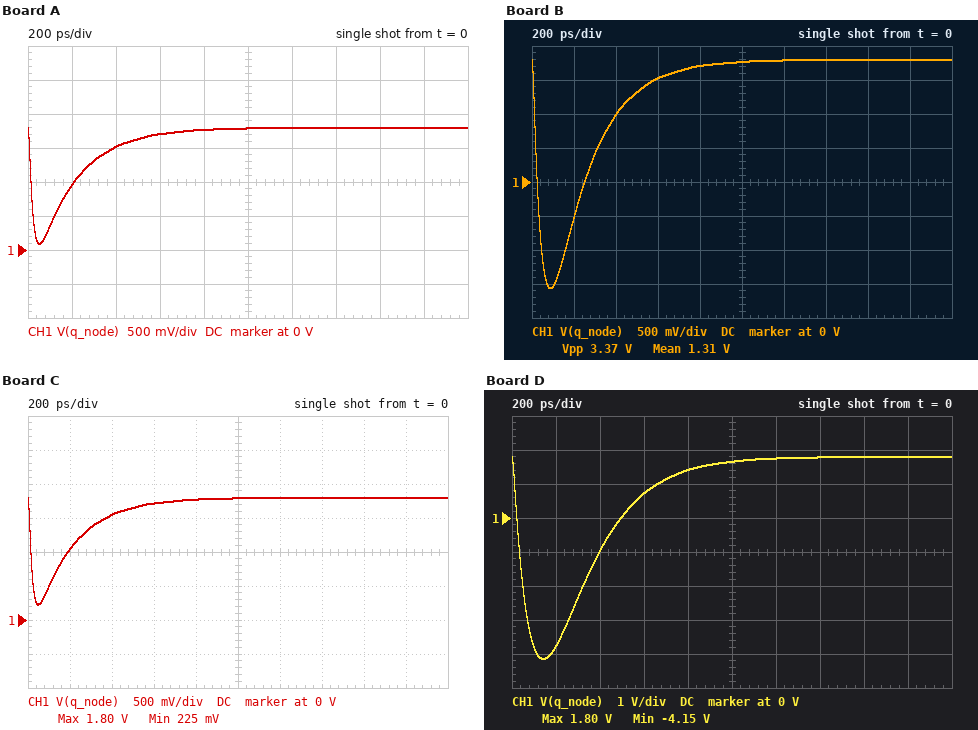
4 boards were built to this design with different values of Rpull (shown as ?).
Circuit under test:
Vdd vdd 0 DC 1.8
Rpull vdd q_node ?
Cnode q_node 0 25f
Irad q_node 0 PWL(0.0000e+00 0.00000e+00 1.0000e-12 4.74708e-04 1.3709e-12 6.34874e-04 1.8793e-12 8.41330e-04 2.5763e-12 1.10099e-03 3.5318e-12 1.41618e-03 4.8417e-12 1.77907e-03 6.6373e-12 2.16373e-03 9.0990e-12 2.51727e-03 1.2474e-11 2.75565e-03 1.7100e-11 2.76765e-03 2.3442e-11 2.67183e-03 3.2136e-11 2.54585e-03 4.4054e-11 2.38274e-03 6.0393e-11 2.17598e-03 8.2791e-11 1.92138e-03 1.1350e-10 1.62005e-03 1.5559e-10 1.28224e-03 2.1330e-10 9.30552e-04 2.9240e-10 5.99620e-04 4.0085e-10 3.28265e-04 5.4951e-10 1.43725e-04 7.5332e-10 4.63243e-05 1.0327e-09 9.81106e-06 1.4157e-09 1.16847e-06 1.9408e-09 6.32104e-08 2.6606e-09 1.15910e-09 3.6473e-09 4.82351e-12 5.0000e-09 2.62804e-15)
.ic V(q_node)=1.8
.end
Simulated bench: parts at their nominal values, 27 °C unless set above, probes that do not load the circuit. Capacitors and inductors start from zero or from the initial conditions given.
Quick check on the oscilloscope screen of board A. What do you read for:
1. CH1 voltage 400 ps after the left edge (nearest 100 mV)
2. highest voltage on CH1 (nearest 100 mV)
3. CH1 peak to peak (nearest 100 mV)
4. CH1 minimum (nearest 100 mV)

1.5 V
1.8 V
1.7 V
100 mV
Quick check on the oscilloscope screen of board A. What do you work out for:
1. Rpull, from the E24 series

750 Ω
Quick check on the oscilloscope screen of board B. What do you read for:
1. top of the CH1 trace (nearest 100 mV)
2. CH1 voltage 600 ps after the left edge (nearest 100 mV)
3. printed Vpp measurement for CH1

1.8 V
1.5 V
3.37 V
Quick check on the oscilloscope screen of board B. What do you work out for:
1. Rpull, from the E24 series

1.8 kΩ
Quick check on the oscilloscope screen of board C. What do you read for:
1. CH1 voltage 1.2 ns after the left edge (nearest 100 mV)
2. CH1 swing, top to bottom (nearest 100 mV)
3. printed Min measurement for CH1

1.8 V
1.6 V
225 mV
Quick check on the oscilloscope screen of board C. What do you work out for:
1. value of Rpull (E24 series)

680 Ω
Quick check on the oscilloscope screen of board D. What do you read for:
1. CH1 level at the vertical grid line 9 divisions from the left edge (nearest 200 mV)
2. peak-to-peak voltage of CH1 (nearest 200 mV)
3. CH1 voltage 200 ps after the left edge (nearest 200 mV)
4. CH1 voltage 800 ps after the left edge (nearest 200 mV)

1.8 V
6.0 V
-3.8 V
1.4 V
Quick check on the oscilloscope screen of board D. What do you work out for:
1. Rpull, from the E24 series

4.3 kΩ
